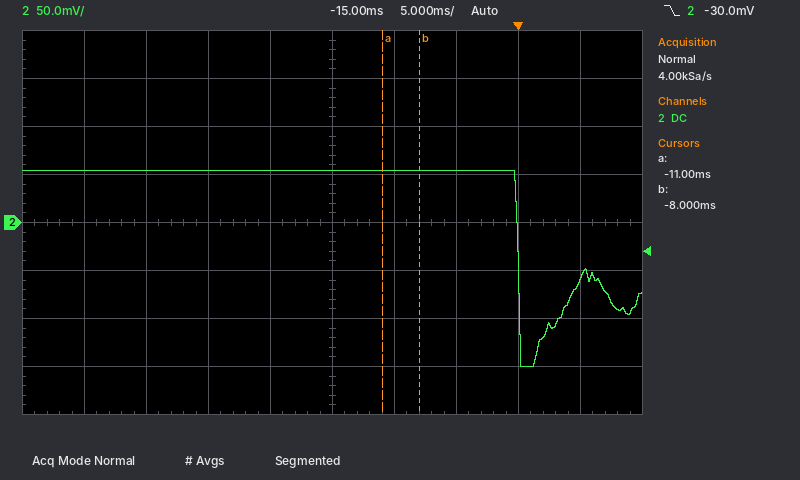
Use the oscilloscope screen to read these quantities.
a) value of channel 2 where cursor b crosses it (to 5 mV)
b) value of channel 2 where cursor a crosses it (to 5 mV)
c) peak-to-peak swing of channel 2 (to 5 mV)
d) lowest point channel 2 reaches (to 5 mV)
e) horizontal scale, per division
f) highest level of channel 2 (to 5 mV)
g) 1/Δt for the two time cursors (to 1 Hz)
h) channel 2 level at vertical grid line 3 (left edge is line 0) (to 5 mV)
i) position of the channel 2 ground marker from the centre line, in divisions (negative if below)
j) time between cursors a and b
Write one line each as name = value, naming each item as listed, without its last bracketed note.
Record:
value of channel 2 where cursor b crosses it = 55 mV
value of channel 2 where cursor a crosses it = 55 mV
peak-to-peak swing of channel 2 = 205 mV
lowest point channel 2 reaches = -150 mV
horizontal scale, per division = 5 ms
highest level of channel 2 = 55 mV
1/Δt for the two time cursors = 333 Hz
channel 2 level at vertical grid line 3 (left edge is line 0) = 55 mV
position of the channel 2 ground marker from the centre line, in divisions = 0.0 div
time between cursors a and b = 3.0 ms
